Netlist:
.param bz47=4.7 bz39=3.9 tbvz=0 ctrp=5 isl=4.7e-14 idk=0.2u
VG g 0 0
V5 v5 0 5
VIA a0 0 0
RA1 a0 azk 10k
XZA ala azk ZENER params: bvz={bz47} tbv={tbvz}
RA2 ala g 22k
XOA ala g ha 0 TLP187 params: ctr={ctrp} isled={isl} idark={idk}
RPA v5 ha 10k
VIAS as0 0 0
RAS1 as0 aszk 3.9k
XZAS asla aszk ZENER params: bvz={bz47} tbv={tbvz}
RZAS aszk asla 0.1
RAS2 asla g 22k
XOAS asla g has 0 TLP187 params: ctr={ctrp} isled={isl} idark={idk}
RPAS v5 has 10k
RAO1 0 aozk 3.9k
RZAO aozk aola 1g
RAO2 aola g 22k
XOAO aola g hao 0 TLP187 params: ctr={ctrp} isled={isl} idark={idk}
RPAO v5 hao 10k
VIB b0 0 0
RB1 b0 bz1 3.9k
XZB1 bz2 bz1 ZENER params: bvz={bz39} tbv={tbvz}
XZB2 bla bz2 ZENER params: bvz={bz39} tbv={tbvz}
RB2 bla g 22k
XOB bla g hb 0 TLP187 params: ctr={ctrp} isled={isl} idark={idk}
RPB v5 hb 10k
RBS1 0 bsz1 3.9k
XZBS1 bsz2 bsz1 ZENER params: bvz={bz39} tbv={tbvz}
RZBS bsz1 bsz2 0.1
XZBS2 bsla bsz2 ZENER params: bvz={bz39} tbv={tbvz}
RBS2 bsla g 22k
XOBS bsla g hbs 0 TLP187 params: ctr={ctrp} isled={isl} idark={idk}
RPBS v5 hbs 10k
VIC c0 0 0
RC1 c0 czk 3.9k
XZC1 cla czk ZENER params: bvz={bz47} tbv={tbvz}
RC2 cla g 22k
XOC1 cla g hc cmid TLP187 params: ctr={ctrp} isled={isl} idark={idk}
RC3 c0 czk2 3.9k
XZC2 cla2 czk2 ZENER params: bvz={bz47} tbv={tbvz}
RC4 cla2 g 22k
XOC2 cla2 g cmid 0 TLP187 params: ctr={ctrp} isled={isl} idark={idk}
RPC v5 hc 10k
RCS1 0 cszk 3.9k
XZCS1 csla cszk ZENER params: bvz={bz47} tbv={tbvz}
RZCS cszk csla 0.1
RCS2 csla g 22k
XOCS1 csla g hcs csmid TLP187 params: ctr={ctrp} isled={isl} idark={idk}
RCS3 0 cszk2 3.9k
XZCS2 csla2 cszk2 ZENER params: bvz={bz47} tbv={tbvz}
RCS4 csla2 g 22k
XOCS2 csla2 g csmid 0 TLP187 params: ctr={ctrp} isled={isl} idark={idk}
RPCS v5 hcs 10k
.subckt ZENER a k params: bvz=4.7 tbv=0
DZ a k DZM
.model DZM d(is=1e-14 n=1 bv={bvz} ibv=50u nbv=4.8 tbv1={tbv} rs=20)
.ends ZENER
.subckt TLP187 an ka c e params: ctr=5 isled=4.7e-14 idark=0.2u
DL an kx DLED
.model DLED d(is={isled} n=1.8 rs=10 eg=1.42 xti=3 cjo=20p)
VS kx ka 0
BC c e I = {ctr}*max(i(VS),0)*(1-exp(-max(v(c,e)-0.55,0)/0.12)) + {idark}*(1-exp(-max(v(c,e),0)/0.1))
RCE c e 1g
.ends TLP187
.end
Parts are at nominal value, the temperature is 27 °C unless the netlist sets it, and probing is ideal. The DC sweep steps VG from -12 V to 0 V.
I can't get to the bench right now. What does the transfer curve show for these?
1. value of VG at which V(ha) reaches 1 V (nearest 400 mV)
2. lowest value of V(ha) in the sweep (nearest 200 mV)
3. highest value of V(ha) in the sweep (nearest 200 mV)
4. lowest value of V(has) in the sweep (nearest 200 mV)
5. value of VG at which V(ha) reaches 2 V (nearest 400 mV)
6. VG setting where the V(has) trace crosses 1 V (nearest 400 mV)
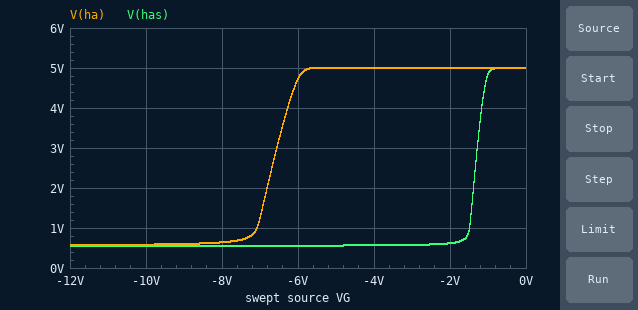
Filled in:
-7.2 V
600 mV
5.0 V
600 mV
-6.8 V
-1.6 V
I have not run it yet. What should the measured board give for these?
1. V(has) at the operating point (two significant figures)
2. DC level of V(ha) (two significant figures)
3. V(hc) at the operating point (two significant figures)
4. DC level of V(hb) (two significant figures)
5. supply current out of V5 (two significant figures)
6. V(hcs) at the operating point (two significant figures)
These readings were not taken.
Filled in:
5.0 V
5.0 V
5.0 V
5.0 V
1.4 µA
5.0 V
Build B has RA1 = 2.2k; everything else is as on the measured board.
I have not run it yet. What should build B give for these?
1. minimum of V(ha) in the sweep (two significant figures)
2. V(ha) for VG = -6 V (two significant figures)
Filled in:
550 mV
2.0 V
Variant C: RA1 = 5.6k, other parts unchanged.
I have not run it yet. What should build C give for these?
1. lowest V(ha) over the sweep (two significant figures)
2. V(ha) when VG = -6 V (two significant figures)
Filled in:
560 mV
4.0 V
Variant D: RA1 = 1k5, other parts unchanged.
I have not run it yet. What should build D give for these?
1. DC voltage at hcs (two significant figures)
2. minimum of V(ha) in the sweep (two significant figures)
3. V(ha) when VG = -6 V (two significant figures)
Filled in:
5.0 V
550 mV
1.0 V
